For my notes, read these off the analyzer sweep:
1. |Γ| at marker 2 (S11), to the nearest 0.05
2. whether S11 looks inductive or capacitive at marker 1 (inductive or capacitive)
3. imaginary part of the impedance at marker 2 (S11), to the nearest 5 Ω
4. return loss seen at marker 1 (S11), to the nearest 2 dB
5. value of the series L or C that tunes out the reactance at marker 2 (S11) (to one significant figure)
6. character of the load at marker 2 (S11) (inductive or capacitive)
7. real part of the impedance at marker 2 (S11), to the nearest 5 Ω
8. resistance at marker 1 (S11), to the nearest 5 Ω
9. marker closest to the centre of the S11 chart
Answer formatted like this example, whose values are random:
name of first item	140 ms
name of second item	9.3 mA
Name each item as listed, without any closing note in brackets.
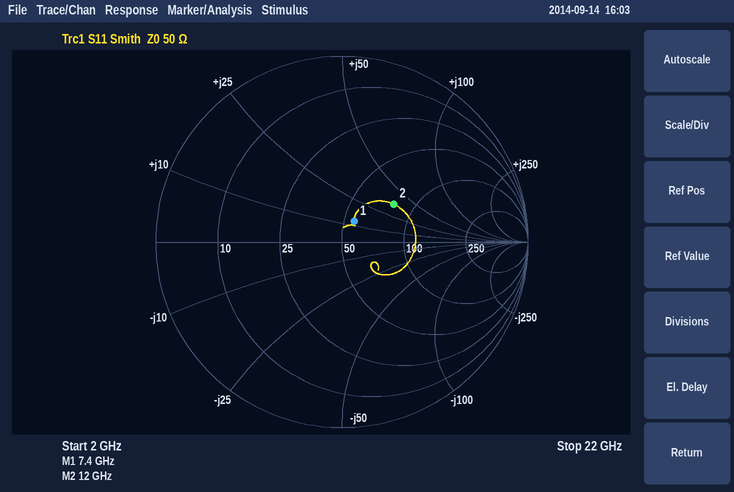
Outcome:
|Γ| at marker 2 (S11), to the nearest 0.05	0.35
whether S11 looks inductive or capacitive at marker 1	inductive
imaginary part of the impedance at marker 2 (S11), to the nearest 5 Ω	+35 Ω
return loss seen at marker 1 (S11), to the nearest 2 dB	18 dB
value of the series L or C that tunes out the reactance at marker 2 (S11)	400 fF
character of the load at marker 2 (S11)	inductive
real part of the impedance at marker 2 (S11), to the nearest 5 Ω	80 Ω
resistance at marker 1 (S11), to the nearest 5 Ω	55 Ω
marker closest to the centre of the S11 chart	marker 1
